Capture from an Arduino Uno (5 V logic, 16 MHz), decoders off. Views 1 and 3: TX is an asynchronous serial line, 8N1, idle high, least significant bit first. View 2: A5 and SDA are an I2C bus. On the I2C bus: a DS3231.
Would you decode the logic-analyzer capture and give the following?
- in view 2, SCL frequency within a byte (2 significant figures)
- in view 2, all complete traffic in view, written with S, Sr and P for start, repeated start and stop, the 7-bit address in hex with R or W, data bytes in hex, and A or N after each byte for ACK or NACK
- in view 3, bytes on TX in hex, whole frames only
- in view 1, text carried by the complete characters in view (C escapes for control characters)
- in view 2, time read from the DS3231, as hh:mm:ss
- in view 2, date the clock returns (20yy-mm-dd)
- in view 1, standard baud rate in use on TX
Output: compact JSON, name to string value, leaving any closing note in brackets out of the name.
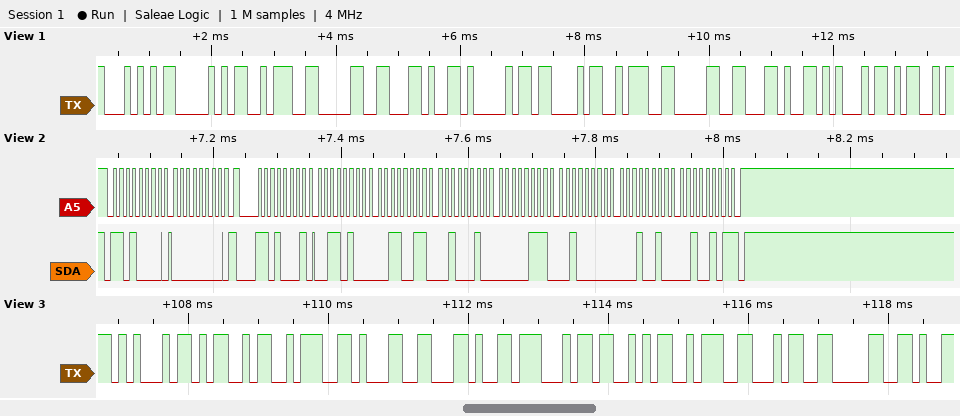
{"in view 2, SCL frequency within a byte": "100 kHz", "in view 2, all complete traffic in view, written with S, Sr and P for start, repeated start and stop, the 7-bit address in hex with R or W, data bytes in hex, and A or N after each byte for ACK or NACK": "S 68W A 00 A Sr 68R A 34 A 33 A 22 A 07 A 20 A 12 A 25 N P", "in view 3, bytes on TX in hex, whole frames only": "45 4D 3A 31 2C 47 53 3A 34 30", "in view 1, text carried by the complete characters in view": "\"TP:0,AC:0,EM\"", "in view 2, time read from the DS3231, as hh:mm:ss": "22:33:34", "in view 2, date the clock returns": "2025-12-20", "in view 1, standard baud rate in use on TX": "9600 baud"}
